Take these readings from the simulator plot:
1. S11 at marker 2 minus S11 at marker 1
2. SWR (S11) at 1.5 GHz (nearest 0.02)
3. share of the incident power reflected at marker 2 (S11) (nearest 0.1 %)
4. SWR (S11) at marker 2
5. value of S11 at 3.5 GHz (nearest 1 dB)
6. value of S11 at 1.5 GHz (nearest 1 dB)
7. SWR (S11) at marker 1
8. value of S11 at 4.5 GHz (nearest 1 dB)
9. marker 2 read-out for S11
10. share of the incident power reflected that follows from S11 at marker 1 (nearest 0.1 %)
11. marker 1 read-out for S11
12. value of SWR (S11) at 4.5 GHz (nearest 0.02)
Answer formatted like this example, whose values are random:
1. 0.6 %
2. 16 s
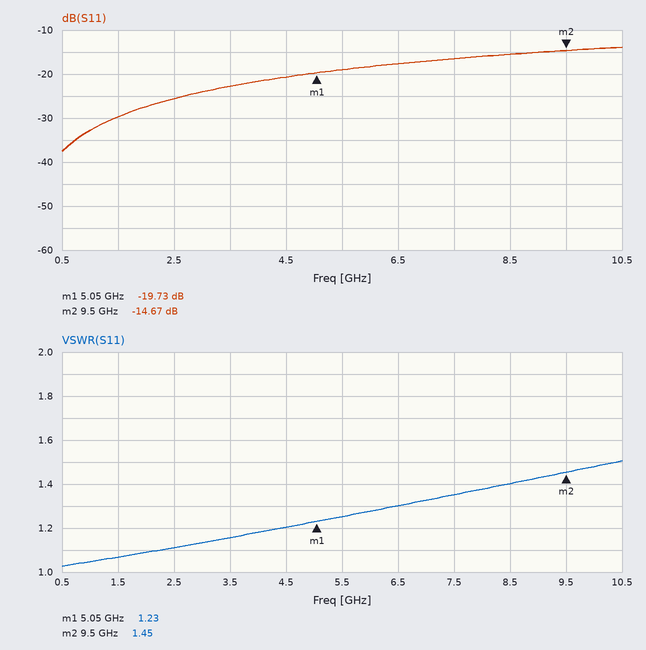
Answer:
1. 5.06 dB
2. 1.06
3. 3.4 %
4. 1.45
5. -23 dB
6. -30 dB
7. 1.23
8. -21 dB
9. -14.67 dB
10. 1.1 %
11. -19.73 dB
12. 1.20
